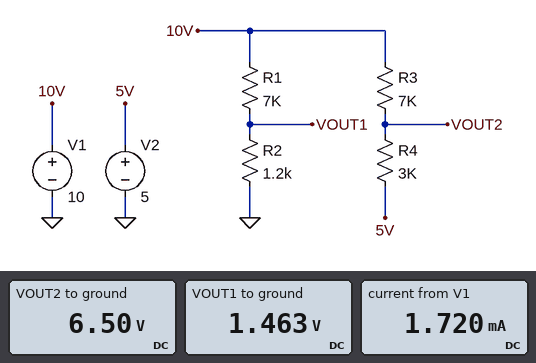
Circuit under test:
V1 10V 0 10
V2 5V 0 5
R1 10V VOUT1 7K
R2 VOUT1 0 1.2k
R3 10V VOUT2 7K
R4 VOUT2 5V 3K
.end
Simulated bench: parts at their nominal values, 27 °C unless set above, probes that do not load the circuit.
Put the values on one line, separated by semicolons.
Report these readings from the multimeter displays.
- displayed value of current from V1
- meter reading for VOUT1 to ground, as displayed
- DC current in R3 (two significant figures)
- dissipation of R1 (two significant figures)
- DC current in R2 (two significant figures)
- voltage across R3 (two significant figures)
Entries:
1.720 mA; 1.463 V; 500 µA; 10 mW; 1.2 mA; 3.5 V
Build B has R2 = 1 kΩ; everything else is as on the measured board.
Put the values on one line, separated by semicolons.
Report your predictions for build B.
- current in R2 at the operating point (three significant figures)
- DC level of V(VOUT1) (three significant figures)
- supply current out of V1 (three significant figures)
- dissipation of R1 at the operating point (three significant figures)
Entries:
1.25 mA; 1.25 V; 1.75 mA; 10.9 mW
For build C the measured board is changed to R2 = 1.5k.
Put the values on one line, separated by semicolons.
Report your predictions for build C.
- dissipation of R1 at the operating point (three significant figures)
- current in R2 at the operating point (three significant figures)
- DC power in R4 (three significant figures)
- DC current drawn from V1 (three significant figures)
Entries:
9.69 mW; 1.18 mA; 750 µW; 1.68 mA
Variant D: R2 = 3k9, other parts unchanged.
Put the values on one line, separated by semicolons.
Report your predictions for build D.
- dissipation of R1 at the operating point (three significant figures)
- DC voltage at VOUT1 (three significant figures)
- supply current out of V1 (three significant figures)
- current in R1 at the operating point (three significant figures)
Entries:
5.89 mW; 3.58 V; 1.42 mA; 917 µA
